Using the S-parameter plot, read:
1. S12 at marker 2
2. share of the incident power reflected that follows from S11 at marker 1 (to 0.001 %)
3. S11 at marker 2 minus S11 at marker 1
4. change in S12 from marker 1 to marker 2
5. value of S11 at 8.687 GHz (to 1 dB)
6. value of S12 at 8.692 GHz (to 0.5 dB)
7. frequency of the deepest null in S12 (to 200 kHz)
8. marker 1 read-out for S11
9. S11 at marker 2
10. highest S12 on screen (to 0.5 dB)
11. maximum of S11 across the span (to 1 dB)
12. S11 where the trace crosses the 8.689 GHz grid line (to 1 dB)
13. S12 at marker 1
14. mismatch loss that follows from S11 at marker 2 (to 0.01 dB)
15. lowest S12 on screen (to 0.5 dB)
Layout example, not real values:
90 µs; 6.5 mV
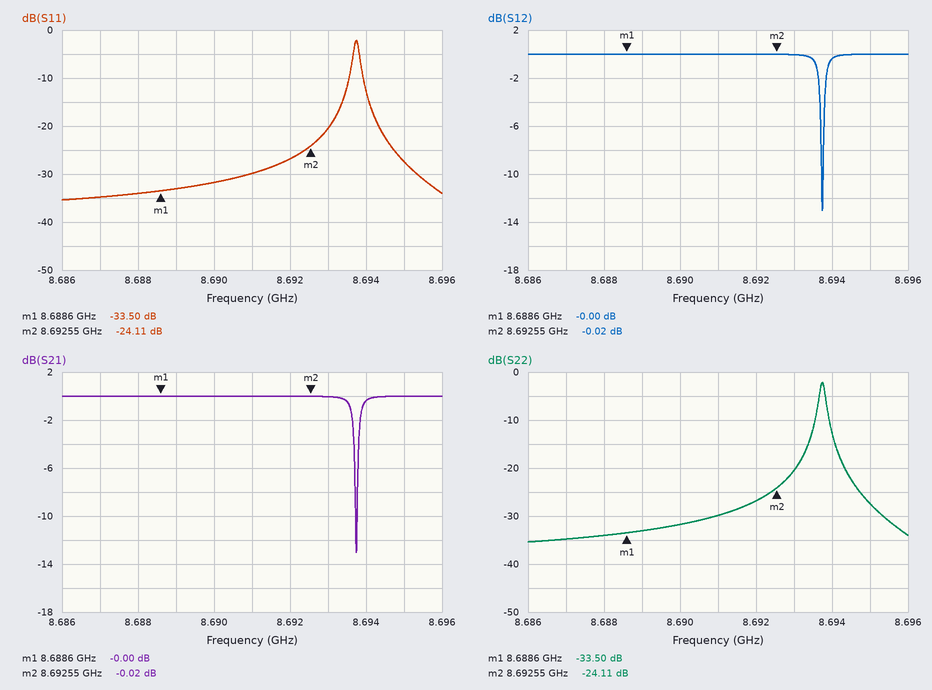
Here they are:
-0.02 dB; 0.045 %; 9.39 dB; -0.02 dB; -35 dB; 0.0 dB; 8.6938 GHz; -33.50 dB; -24.11 dB; 0.0 dB; -2 dB; -33 dB; -0.00 dB; 0.02 dB; -13.0 dB
